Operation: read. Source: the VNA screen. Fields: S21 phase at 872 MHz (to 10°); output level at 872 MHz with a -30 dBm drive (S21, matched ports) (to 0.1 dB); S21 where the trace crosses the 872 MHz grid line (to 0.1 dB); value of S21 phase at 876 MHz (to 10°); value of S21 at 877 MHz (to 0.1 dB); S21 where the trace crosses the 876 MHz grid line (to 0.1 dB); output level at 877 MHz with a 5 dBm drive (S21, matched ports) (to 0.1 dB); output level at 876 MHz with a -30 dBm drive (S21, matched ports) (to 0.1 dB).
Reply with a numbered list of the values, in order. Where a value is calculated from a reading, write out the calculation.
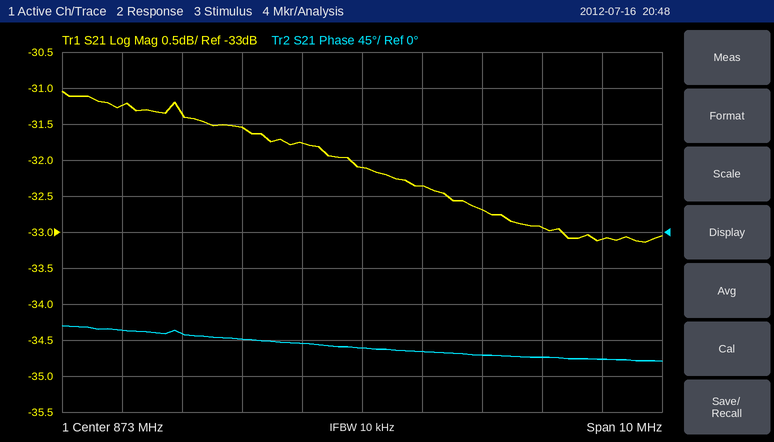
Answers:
1. -140°
2. -30 dBm + (-31.8 dB) = -61.8 dBm
3. -31.8 dB
4. -160°
5. -33.1 dB
6. -32.9 dB
7. 5 dBm + (-33.1 dB) = -28.1 dBm
8. -30 dBm + (-32.9 dB) = -62.9 dBm
